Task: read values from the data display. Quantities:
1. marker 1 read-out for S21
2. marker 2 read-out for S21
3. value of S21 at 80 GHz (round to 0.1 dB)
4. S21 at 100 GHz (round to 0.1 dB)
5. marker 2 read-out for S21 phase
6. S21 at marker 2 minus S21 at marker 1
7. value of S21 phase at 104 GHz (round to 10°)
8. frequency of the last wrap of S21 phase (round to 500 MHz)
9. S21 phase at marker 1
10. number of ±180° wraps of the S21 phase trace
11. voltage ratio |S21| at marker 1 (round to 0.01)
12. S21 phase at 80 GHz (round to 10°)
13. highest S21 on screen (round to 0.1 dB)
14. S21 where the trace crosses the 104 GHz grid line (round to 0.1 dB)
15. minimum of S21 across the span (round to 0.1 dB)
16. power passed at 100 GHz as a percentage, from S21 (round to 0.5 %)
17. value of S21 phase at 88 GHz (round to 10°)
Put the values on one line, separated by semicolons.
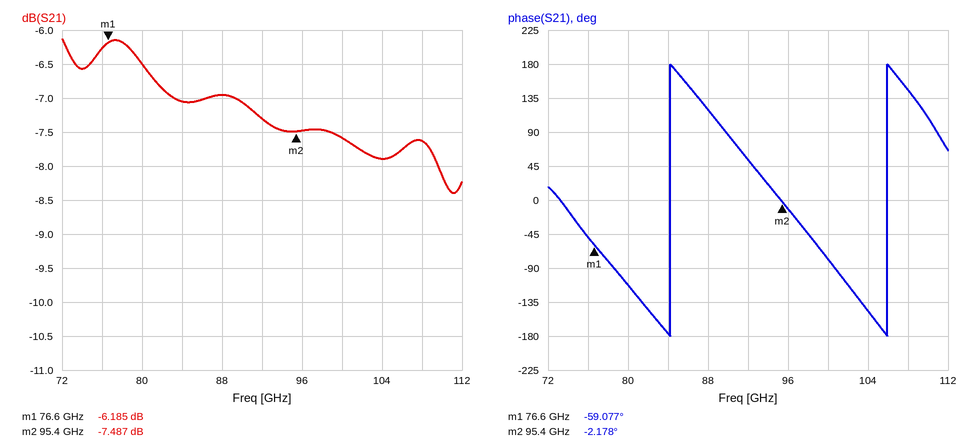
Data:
-6.185 dB; -7.487 dB; -6.5 dB; -7.6 dB; -2.178°; -1.302 dB; -150°; 106.0 GHz; -59.077°; 2; 0.49; -110°; -6.1 dB; -7.9 dB; -8.4 dB; 17.5 %; 120°
